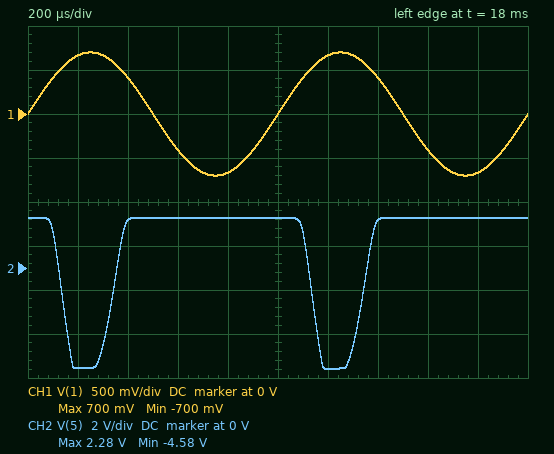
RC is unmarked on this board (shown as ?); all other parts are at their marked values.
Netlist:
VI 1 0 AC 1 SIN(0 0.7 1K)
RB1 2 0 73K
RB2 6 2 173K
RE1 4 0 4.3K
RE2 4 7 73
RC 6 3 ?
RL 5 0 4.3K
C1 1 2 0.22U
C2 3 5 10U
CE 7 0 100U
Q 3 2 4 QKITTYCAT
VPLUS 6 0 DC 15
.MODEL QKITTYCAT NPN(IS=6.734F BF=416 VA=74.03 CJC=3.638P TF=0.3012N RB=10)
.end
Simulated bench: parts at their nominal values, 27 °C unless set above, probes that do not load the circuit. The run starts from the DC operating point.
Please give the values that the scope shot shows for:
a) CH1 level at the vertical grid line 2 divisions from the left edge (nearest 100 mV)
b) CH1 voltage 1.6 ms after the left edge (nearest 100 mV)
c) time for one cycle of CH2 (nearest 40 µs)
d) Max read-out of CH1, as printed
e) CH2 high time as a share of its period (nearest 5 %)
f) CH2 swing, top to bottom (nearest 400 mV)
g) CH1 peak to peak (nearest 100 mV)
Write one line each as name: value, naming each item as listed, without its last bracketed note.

CH1 level at the vertical grid line 2 divisions from the left edge: 400 mV
CH1 voltage 1.6 ms after the left edge: -400 mV
time for one cycle of CH2: 1.00 ms
Max read-out of CH1, as printed: 700 mV
CH2 high time as a share of its period: 80 %
CH2 swing, top to bottom: 6.8 V
CH1 peak to peak: 1.4 V
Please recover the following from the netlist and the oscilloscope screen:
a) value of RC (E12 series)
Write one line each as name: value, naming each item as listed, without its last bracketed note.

value of RC: 8.2 kΩ
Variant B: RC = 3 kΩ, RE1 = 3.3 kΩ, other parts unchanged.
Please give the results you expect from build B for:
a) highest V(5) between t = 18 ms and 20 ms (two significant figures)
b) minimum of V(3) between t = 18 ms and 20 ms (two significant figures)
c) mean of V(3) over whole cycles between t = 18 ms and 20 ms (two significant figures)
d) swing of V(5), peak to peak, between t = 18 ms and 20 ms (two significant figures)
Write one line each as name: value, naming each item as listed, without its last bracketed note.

highest V(5) between t = 18 ms and 20 ms: 2.1 V
minimum of V(3) between t = 18 ms and 20 ms: 4.1 V
mean of V(3) over whole cycles between t = 18 ms and 20 ms: 11 V
swing of V(5), peak to peak, between t = 18 ms and 20 ms: 9.4 V
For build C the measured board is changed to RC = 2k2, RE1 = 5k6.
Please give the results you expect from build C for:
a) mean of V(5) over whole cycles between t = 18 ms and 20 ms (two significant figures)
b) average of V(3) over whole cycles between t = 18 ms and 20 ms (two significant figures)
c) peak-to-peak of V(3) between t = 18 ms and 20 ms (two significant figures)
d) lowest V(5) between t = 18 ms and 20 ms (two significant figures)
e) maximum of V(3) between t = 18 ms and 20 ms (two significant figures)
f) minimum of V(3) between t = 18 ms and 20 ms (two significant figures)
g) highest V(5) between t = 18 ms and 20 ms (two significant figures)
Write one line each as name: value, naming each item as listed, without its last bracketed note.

mean of V(5) over whole cycles between t = 18 ms and 20 ms: -660 mV
average of V(3) over whole cycles between t = 18 ms and 20 ms: 12 V
peak-to-peak of V(3) between t = 18 ms and 20 ms: 8.0 V
lowest V(5) between t = 18 ms and 20 ms: -6.7 V
maximum of V(3) between t = 18 ms and 20 ms: 14 V
minimum of V(3) between t = 18 ms and 20 ms: 6.3 V
highest V(5) between t = 18 ms and 20 ms: 1.3 V
